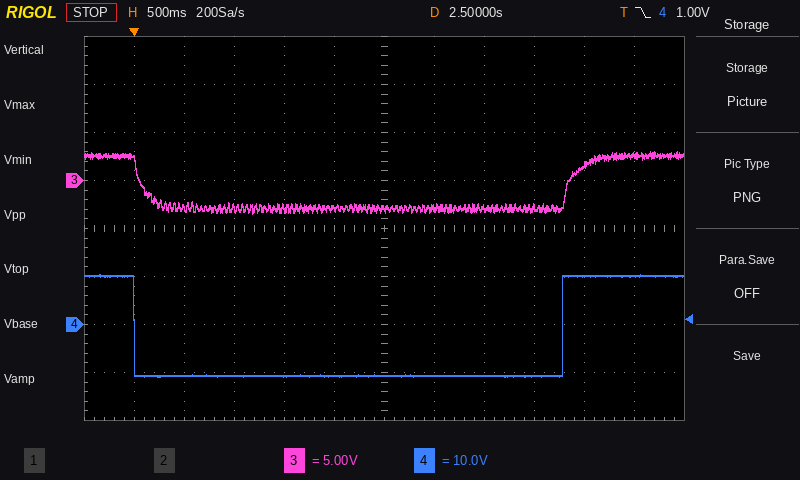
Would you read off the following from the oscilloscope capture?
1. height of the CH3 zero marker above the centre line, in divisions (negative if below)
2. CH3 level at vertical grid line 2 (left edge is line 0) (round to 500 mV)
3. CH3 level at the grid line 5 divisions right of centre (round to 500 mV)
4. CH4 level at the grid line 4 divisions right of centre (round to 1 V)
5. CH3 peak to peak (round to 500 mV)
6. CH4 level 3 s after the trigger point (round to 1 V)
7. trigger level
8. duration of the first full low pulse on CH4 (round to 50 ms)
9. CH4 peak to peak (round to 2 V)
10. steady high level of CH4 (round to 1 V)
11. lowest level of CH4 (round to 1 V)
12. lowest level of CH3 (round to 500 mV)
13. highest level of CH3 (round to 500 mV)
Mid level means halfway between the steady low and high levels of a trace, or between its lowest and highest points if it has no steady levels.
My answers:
+1.0 div
-3.0 V
2.5 V
10 V
6.5 V
-11 V
1.00 V
4.30 s
22 V
10 V
-11 V
-3.5 V
3.0 V
